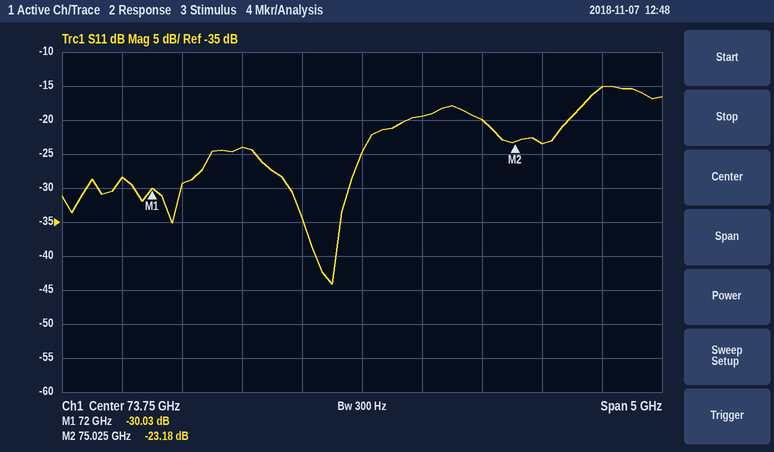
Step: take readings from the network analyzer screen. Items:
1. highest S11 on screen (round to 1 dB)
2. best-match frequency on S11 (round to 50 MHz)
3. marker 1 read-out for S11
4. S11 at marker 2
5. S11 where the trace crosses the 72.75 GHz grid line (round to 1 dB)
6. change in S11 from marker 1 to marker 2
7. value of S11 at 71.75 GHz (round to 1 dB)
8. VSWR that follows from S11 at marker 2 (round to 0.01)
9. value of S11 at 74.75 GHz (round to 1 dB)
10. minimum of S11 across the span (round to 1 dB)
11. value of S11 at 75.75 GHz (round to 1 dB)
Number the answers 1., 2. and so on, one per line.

1. -15 dB
2. 73.50 GHz
3. -30.03 dB
4. -23.18 dB
5. -24 dB
6. 6.85 dB
7. -28 dB
8. 1.15
9. -20 dB
10. -44 dB
11. -15 dB
